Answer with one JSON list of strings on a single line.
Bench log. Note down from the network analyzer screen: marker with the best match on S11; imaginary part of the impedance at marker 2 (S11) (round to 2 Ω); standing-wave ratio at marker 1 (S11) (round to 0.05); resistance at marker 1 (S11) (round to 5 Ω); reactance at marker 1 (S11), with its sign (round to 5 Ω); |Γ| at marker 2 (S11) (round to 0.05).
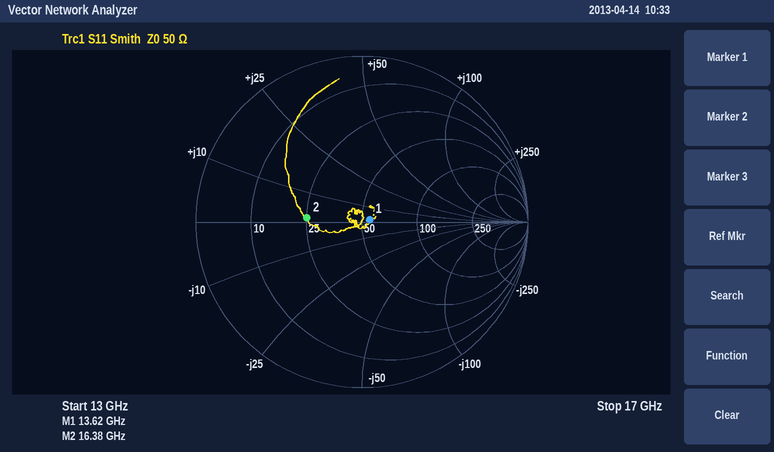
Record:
["marker 1", "+2 Ω", "1.10", "55 Ω", "0 Ω", "0.35"]
